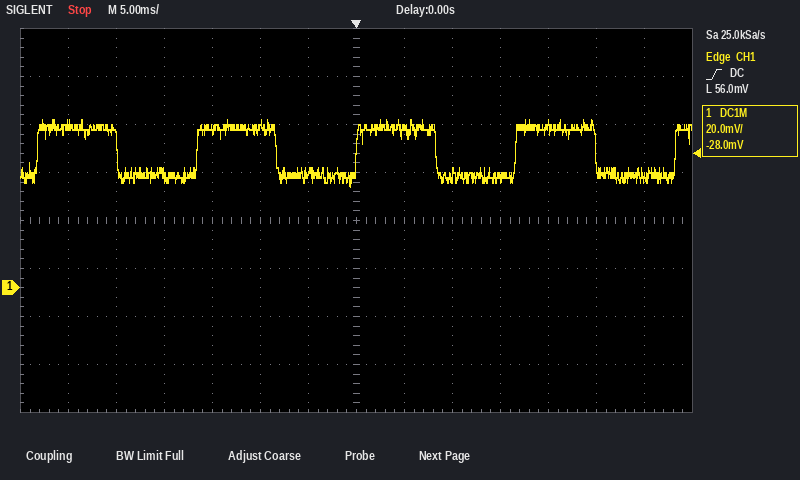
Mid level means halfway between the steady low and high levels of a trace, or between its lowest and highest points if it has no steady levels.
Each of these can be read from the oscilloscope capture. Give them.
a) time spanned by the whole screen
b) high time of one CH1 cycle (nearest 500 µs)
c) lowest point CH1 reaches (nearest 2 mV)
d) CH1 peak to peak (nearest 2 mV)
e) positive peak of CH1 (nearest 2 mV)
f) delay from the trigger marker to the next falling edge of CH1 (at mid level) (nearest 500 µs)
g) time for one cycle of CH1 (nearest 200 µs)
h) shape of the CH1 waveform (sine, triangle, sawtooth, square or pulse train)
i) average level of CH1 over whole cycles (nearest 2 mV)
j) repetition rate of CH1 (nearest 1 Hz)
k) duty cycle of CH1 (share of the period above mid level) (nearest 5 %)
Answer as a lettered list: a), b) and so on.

a) 70 ms
b) 8.5 ms
c) 42 mV
d) 28 mV
e) 70 mV
f) 8.5 ms
g) 16.6 ms
h) square
i) 56 mV
j) 60 Hz
k) 50 %
